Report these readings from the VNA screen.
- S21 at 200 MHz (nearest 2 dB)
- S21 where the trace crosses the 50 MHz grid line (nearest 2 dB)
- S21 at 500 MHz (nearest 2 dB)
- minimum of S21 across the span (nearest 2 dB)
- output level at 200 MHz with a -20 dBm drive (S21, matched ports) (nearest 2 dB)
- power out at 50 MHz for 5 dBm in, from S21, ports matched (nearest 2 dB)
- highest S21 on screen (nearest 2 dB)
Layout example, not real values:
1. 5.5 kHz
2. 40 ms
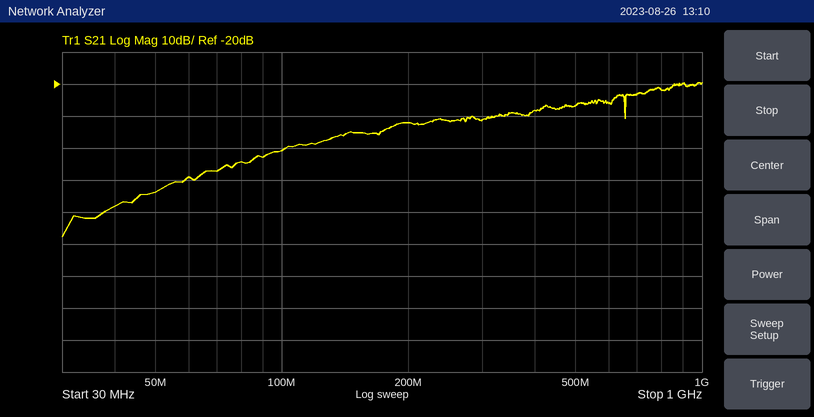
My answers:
1. -32 dB
2. -54 dB
3. -26 dB
4. -68 dB
5. -52 dBm
6. -48 dBm
7. -20 dB
